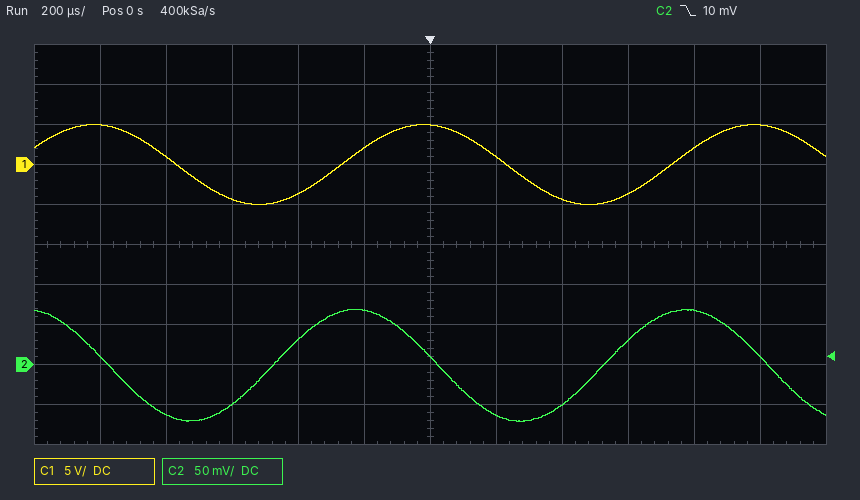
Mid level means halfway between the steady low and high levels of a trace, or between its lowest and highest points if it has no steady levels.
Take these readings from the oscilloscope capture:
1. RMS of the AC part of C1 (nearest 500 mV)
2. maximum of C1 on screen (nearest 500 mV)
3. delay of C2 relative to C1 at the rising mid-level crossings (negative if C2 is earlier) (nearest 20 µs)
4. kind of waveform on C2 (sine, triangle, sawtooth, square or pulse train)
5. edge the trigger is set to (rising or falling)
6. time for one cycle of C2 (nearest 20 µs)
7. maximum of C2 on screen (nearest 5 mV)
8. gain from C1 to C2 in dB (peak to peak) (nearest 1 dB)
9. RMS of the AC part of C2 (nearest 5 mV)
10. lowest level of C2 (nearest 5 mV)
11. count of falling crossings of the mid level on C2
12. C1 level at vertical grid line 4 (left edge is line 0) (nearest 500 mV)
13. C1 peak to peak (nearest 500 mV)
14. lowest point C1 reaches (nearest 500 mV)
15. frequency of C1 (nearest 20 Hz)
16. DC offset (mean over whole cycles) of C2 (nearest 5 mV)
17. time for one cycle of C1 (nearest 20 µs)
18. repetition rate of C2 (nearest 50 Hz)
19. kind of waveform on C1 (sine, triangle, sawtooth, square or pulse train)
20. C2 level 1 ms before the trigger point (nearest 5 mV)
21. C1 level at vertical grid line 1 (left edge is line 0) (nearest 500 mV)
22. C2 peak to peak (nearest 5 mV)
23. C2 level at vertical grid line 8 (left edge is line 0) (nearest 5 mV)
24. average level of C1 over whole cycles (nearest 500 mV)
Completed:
3.5 V
5.0 V
-200 µs
sine
falling
1.00 ms
70 mV
-37 dB
50 mV
-70 mV
3
-3.5 V
10.0 V
-5.0 V
1.00 kHz
0 mV
1.00 ms
1.00 kHz
sine
10 mV
5.0 V
140 mV
-50 mV
0.0 V
